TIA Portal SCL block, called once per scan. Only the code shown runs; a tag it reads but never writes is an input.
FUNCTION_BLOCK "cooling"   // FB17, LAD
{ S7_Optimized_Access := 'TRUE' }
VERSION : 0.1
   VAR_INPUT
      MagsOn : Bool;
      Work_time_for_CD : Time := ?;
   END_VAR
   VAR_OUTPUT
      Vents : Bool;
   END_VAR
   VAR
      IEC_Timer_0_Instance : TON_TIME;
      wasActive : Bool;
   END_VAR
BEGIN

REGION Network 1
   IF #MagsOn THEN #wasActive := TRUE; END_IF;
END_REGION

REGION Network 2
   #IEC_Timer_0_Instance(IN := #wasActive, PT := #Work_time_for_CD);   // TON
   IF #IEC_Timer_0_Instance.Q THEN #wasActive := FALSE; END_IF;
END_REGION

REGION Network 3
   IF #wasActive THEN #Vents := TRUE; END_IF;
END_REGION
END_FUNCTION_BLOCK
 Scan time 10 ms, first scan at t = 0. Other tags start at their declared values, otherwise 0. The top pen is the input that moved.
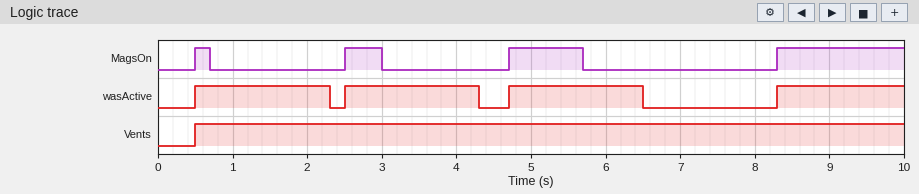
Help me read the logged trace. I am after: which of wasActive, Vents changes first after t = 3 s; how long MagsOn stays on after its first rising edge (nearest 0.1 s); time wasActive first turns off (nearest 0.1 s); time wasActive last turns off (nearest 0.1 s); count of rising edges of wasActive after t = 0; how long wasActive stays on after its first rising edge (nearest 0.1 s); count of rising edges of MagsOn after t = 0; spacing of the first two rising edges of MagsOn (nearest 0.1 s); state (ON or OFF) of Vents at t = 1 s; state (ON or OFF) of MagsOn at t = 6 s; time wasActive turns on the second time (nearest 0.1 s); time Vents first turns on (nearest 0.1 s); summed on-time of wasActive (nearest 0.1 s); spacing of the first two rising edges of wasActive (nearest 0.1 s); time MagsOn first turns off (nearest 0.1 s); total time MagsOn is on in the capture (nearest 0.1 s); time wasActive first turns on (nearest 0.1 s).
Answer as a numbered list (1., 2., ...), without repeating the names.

1. wasActive
2. 0.2 s
3. 2.3 s
4. 6.5 s
5. 4
6. 1.8 s
7. 4
8. 2.0 s
9. ON
10. OFF
11. 2.5 s
12. 0.5 s
13. 7.1 s
14. 2.0 s
15. 0.7 s
16. 3.4 s
17. 0.5 s
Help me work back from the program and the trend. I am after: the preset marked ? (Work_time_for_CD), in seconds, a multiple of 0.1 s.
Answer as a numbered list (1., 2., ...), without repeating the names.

1. 1.8 s
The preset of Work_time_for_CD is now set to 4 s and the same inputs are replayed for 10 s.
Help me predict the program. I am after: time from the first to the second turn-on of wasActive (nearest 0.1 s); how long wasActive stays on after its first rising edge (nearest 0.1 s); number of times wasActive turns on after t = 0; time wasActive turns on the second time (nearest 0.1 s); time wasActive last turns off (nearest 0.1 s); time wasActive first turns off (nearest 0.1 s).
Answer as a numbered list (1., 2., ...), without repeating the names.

1. 4.2 s
2. 4.0 s
3. 2
4. 4.7 s
5. 8.7 s
6. 4.5 s
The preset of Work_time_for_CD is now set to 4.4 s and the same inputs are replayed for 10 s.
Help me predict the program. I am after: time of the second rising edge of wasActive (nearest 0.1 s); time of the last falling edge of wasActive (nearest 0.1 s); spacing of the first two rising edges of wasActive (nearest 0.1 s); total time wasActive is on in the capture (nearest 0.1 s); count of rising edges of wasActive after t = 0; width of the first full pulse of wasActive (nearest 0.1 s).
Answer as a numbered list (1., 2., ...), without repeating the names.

1. 8.3 s
2. 4.9 s
3. 7.8 s
4. 6.1 s
5. 2
6. 4.4 s
